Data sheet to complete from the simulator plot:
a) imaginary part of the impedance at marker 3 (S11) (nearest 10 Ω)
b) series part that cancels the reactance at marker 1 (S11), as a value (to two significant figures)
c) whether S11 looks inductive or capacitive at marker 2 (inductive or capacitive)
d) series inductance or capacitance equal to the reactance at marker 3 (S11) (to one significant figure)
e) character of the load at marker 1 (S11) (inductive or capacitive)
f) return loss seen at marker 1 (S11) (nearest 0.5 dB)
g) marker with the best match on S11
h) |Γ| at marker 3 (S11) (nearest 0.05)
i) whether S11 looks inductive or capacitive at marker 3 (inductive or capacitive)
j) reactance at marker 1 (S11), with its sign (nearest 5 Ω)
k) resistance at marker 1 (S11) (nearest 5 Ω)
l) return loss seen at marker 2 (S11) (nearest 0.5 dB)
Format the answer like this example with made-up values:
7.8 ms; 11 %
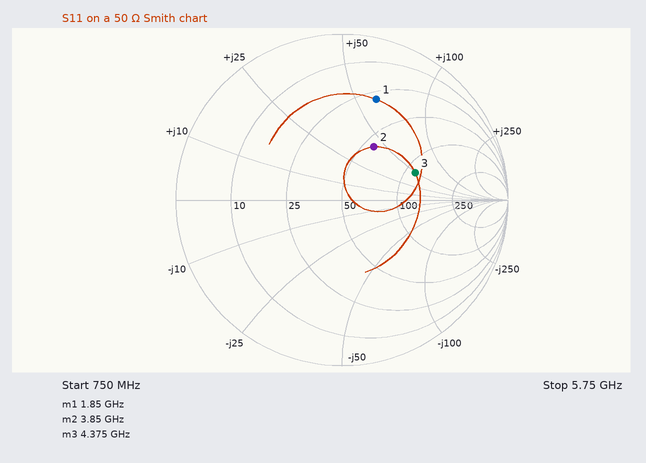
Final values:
+50 Ω; 1.4 pF; inductive; 2 nH; inductive; 4.0 dB; marker 2; 0.45; inductive; +60 Ω; 30 Ω; 8.5 dB
